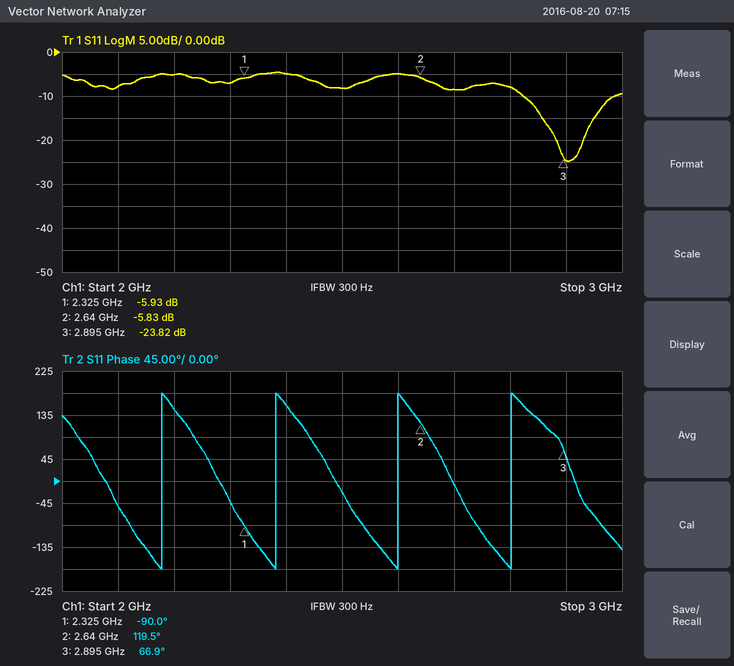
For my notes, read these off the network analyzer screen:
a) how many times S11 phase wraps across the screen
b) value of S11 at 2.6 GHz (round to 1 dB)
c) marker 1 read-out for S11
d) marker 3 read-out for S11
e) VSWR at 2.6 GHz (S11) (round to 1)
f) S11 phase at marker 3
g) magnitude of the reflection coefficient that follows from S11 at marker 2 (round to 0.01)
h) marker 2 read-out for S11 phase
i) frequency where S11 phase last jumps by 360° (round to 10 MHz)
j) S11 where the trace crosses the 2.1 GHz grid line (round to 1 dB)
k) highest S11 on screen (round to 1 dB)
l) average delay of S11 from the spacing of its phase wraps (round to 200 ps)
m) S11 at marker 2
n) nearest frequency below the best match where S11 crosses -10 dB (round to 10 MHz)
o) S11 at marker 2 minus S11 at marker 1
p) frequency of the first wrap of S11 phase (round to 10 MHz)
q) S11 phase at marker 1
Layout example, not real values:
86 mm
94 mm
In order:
4
-5 dB
-5.93 dB
-23.82 dB
4
66.9°
0.51
119.5°
2.80 GHz
-8 dB
-5 dB
4.8 ns
-5.83 dB
2.82 GHz
0.10 dB
2.18 GHz
-90.0°
